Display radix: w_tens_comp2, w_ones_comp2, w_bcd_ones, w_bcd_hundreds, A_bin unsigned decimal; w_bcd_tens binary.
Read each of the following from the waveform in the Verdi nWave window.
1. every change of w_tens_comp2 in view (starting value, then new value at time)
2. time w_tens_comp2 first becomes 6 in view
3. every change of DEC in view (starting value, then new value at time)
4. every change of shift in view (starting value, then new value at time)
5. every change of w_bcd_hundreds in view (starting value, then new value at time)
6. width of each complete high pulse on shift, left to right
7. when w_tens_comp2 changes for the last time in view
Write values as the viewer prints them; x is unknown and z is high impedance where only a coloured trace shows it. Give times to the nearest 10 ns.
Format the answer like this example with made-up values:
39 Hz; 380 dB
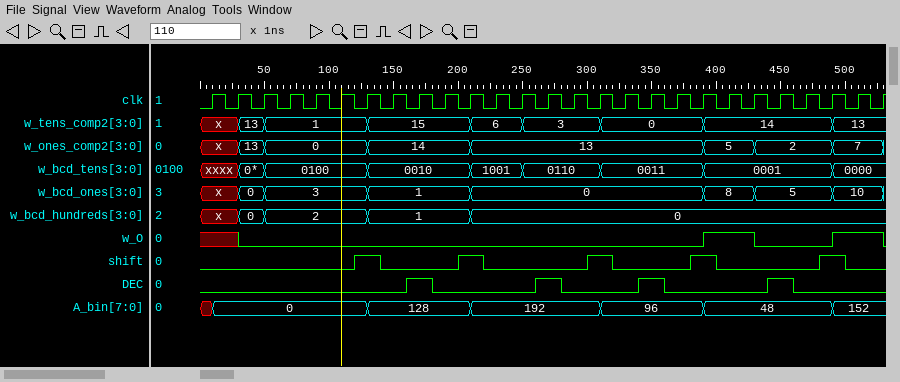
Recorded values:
x, 13 at 30 ns, 1 at 50 ns, 15 at 130 ns, 6 at 210 ns, 3 at 250 ns, 0 at 310 ns, 14 at 390 ns, 13 at 490 ns; 210 ns; 0, 1 at 160 ns, 0 at 180 ns, 1 at 260 ns, 0 at 280 ns, 1 at 340 ns, 0 at 360 ns, 1 at 440 ns, 0 at 460 ns; 0, 1 at 120 ns, 0 at 140 ns, 1 at 200 ns, 0 at 220 ns, 1 at 300 ns, 0 at 320 ns, 1 at 380 ns, 0 at 400 ns, 1 at 480 ns, 0 at 500 ns; x, 0 at 30 ns, 2 at 50 ns, 1 at 130 ns, 0 at 210 ns; 20 ns, 20 ns, 20 ns, 20 ns, 20 ns; 490 ns
